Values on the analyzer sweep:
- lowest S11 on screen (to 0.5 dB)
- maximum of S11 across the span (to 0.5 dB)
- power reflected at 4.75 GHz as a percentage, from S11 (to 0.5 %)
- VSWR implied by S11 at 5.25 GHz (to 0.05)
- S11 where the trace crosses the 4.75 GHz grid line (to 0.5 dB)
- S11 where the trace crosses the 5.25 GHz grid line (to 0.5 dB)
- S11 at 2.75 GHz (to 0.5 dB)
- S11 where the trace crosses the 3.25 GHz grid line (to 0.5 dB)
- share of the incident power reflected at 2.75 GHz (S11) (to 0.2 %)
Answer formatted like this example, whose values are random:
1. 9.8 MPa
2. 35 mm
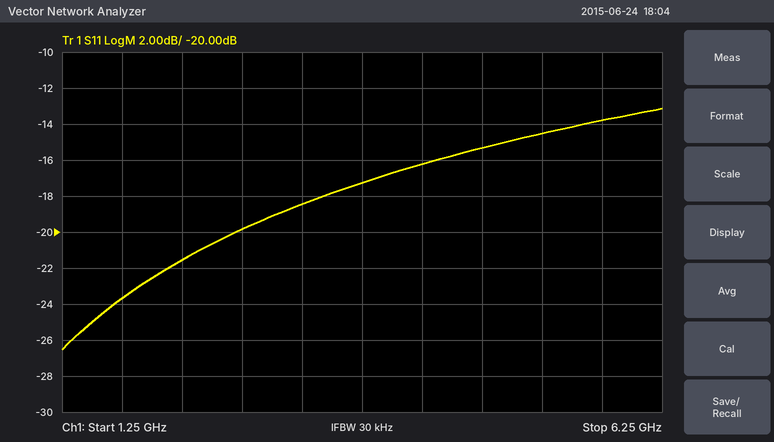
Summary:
1. -26.5 dB
2. -13.0 dB
3. 3.0 %
4. 1.45
5. -15.5 dB
6. -14.5 dB
7. -20.0 dB
8. -18.5 dB
9. 1.0 %
